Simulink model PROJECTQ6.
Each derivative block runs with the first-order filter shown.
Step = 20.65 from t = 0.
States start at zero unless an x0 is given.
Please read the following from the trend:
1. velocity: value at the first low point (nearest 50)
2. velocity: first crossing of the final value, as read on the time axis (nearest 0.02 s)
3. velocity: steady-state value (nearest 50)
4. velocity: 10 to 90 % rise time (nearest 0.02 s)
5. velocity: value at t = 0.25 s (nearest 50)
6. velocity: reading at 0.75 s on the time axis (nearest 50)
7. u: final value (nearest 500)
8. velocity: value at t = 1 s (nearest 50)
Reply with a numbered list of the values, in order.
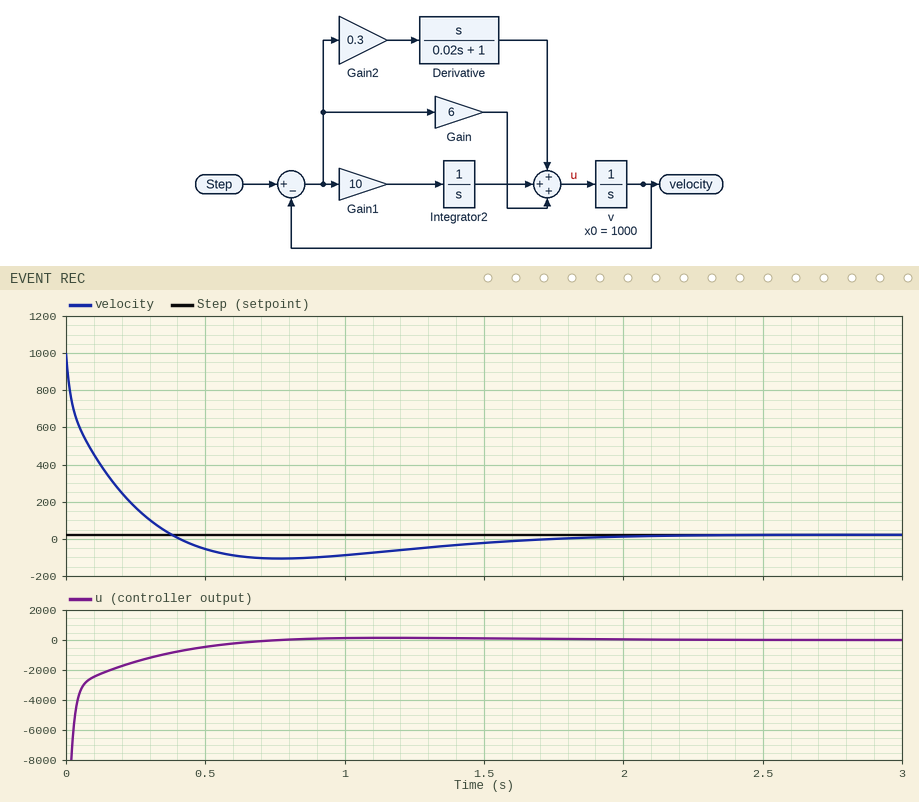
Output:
1. -100
2. 0.38 s
3. 0
4. 0.28 s
5. 150
6. -100
7. 0
8. -100
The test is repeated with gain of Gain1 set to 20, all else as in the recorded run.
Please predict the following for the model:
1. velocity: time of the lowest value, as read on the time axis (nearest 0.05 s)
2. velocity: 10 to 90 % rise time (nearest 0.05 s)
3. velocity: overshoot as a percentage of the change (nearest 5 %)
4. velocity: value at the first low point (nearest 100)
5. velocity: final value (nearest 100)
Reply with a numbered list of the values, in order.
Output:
1. 0.60 s
2. 0.25 s
3. 20 %
4. -200
5. 0
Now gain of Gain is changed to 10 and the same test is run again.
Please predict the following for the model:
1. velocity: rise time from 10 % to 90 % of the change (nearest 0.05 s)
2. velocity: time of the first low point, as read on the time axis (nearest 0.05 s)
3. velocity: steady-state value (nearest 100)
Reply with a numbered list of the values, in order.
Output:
1. 0.20 s
2. 0.65 s
3. 0
